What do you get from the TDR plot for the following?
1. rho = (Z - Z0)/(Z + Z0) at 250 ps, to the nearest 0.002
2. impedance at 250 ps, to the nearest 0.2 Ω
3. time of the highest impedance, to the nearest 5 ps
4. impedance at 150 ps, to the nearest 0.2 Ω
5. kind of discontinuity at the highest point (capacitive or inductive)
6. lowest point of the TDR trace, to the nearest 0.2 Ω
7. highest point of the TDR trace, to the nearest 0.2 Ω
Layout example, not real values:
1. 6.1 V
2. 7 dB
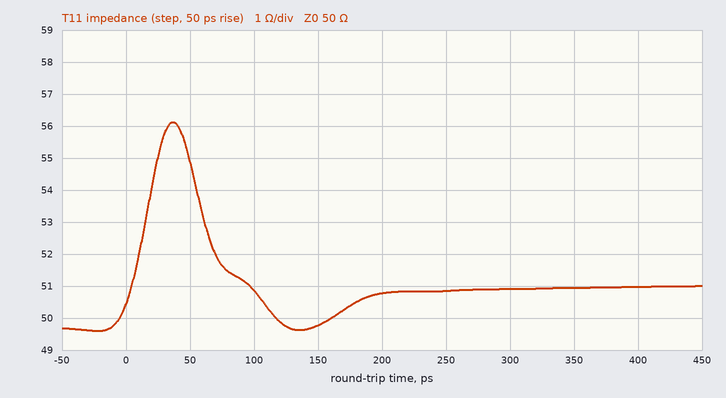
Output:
1. +0.008
2. 50.8 Ω
3. 35 ps
4. 49.8 Ω
5. inductive
6. 49.6 Ω
7. 56.2 Ω
